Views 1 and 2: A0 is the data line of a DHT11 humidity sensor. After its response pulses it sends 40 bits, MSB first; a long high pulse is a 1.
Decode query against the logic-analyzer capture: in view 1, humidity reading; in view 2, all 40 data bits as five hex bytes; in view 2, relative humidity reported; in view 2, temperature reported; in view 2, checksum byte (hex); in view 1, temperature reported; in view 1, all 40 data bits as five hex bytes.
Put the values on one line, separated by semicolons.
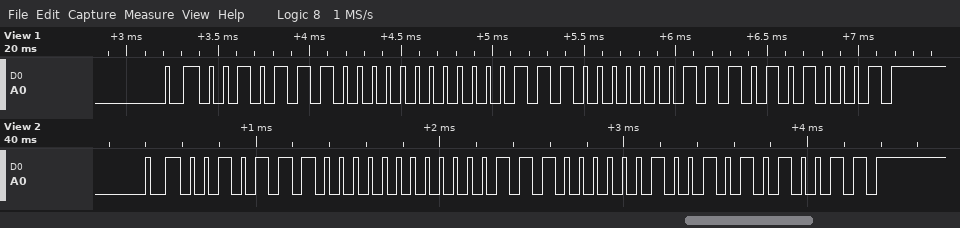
46 %; 2E 00 1C 09 53; 46 %; 28.9 °C; 0x53; 28.7 °C; 2E 00 1C 07 51
